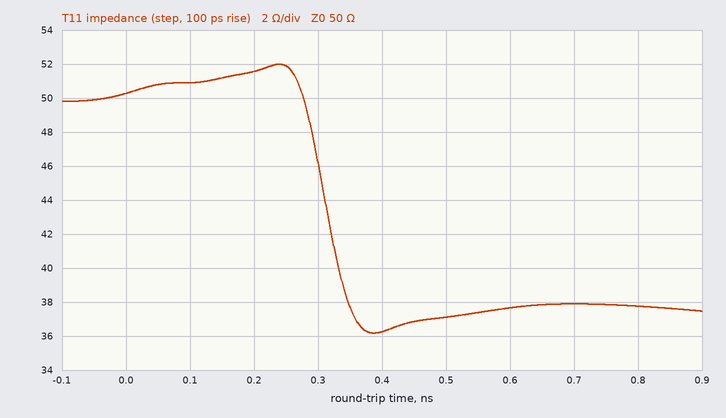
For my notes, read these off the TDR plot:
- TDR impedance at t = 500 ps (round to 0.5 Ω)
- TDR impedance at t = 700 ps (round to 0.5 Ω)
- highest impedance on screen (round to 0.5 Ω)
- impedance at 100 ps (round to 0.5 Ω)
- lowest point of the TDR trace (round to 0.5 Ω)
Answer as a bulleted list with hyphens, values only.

- 37.0 Ω
- 38.0 Ω
- 52.0 Ω
- 51.0 Ω
- 36.0 Ω
